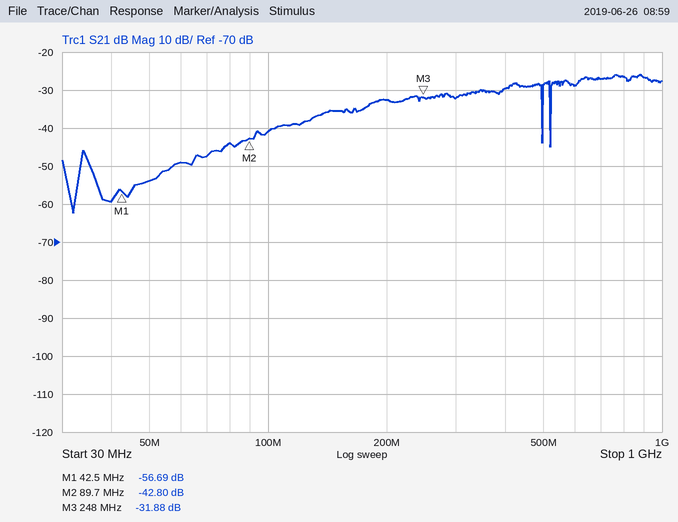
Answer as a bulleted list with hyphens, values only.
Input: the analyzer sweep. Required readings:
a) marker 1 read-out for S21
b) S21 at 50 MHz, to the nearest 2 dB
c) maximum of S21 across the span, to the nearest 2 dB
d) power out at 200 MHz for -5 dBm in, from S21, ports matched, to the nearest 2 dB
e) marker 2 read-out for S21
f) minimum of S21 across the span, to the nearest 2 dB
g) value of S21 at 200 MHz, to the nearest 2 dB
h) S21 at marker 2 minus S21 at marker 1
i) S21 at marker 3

- -56.69 dB
- -54 dB
- -26 dB
- -38 dBm
- -42.80 dB
- -62 dB
- -32 dB
- 13.89 dB
- -31.88 dB
